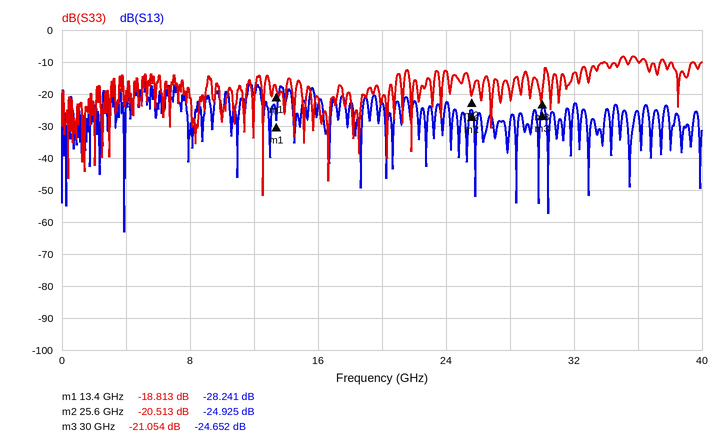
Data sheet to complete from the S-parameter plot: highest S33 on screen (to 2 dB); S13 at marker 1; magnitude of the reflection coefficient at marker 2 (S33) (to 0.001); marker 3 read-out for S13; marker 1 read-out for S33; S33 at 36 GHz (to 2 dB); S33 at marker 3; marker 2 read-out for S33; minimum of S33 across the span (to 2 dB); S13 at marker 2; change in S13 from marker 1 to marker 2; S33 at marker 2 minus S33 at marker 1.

-8 dB
-28.241 dB
0.094
-24.652 dB
-18.813 dB
-10 dB
-21.054 dB
-20.513 dB
-52 dB
-24.925 dB
3.316 dB
-1.700 dB
